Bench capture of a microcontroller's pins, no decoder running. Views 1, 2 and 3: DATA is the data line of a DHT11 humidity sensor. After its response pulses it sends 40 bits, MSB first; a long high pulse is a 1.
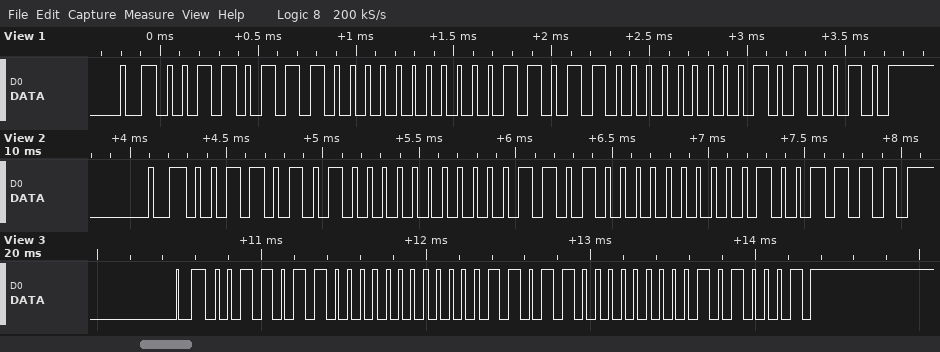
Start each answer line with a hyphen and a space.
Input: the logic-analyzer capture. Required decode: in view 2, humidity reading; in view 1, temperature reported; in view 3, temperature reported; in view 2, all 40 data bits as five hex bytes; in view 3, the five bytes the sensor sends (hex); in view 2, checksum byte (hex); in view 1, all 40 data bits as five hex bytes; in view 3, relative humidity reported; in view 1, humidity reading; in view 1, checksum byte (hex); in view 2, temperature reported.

- 53 %
- 27.0 °C
- 27.0 °C
- 35 00 1A 00 4F
- 36 00 1B 00 51
- 0x4F
- 37 00 1B 00 52
- 54 %
- 55 %
- 0x52
- 26.0 °C
